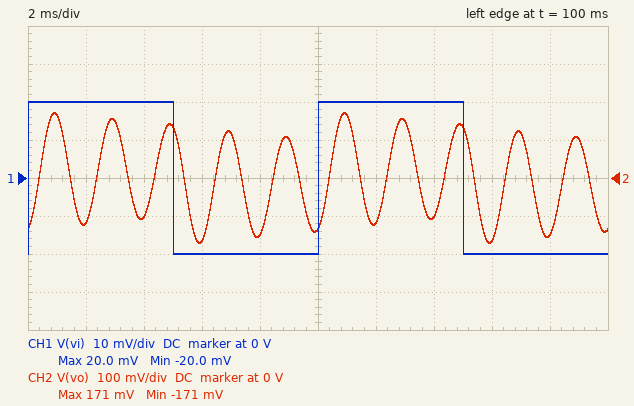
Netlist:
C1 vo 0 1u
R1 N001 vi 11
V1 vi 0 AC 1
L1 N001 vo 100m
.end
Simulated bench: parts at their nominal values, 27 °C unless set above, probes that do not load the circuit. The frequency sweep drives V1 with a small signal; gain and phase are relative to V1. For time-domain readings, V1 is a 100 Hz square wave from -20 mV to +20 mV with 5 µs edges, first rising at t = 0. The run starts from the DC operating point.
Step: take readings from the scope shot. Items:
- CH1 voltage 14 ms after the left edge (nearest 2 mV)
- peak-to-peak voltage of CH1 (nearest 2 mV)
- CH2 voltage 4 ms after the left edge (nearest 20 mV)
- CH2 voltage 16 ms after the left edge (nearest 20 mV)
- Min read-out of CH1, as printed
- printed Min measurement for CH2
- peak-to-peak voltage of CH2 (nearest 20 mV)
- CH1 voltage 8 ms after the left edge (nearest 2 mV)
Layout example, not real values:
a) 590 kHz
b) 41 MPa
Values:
a) 20 mV
b) 40 mV
c) -100 mV
d) -160 mV
e) -20.0 mV
f) -171 mV
g) 340 mV
h) -20 mV
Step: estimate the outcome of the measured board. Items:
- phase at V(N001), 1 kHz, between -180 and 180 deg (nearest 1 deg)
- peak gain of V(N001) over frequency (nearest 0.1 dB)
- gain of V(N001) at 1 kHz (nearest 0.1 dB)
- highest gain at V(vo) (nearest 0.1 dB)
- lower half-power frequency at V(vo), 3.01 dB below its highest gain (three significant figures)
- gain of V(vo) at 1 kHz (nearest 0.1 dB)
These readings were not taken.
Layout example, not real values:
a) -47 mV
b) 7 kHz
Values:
a) 1 deg
b) 0 dB
c) 0 dB
d) 29.2 dB
e) 494 Hz
f) -9.4 dB
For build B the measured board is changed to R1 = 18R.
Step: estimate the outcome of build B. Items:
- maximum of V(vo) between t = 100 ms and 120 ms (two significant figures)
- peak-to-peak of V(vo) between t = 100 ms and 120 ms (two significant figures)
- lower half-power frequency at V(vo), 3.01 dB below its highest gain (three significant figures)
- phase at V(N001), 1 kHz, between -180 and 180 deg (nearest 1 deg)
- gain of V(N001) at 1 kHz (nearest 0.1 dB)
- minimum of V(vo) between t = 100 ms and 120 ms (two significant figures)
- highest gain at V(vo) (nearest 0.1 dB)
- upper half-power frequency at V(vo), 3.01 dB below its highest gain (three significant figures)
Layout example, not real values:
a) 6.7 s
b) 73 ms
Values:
a) 120 mV
b) 240 mV
c) 488 Hz
d) 2 deg
e) 0 dB
f) -120 mV
g) 24.9 dB
h) 517 Hz
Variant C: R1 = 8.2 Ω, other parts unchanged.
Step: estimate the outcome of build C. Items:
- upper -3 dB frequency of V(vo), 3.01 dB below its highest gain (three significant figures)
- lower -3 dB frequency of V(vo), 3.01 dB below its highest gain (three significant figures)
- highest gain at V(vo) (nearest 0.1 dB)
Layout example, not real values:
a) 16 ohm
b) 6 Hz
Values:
a) 510 Hz
b) 497 Hz
c) 31.7 dB
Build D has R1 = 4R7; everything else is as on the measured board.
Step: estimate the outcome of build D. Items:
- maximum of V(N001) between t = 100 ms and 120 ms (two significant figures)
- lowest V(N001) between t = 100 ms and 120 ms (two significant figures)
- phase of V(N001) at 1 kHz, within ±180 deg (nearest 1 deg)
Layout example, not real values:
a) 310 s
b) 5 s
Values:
a) 24 mV
b) -24 mV
c) 1 deg
